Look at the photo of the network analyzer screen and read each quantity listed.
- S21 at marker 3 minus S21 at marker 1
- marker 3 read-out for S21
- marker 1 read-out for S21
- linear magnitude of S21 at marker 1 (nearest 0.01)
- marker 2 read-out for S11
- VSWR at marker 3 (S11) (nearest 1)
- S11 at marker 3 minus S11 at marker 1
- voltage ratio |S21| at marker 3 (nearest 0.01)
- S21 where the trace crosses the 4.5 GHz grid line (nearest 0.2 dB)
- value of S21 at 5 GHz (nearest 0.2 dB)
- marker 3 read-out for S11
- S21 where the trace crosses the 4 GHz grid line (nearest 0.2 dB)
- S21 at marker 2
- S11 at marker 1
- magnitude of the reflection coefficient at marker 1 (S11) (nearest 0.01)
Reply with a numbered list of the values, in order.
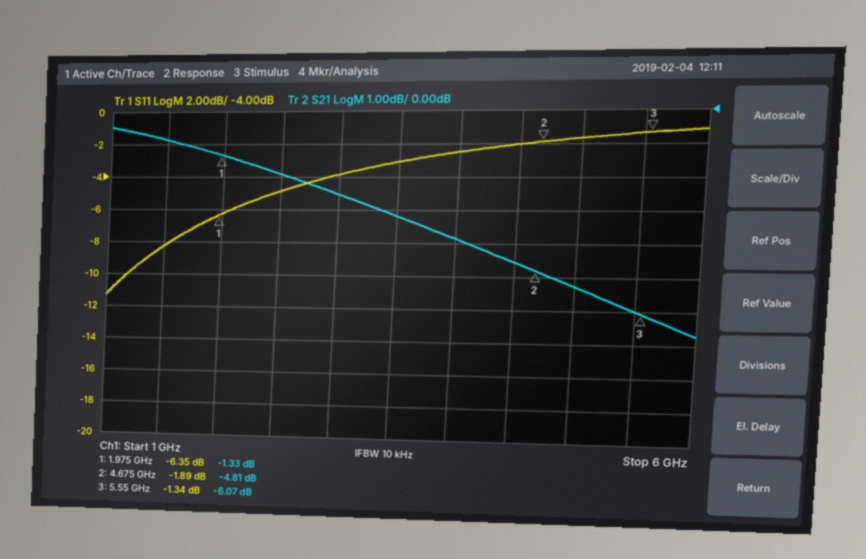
1. -4.74 dB
2. -6.07 dB
3. -1.33 dB
4. 0.86
5. -1.89 dB
6. 13
7. 5.01 dB
8. 0.50
9. -4.6 dB
10. -5.2 dB
11. -1.34 dB
12. -3.8 dB
13. -4.81 dB
14. -6.35 dB
15. 0.48
